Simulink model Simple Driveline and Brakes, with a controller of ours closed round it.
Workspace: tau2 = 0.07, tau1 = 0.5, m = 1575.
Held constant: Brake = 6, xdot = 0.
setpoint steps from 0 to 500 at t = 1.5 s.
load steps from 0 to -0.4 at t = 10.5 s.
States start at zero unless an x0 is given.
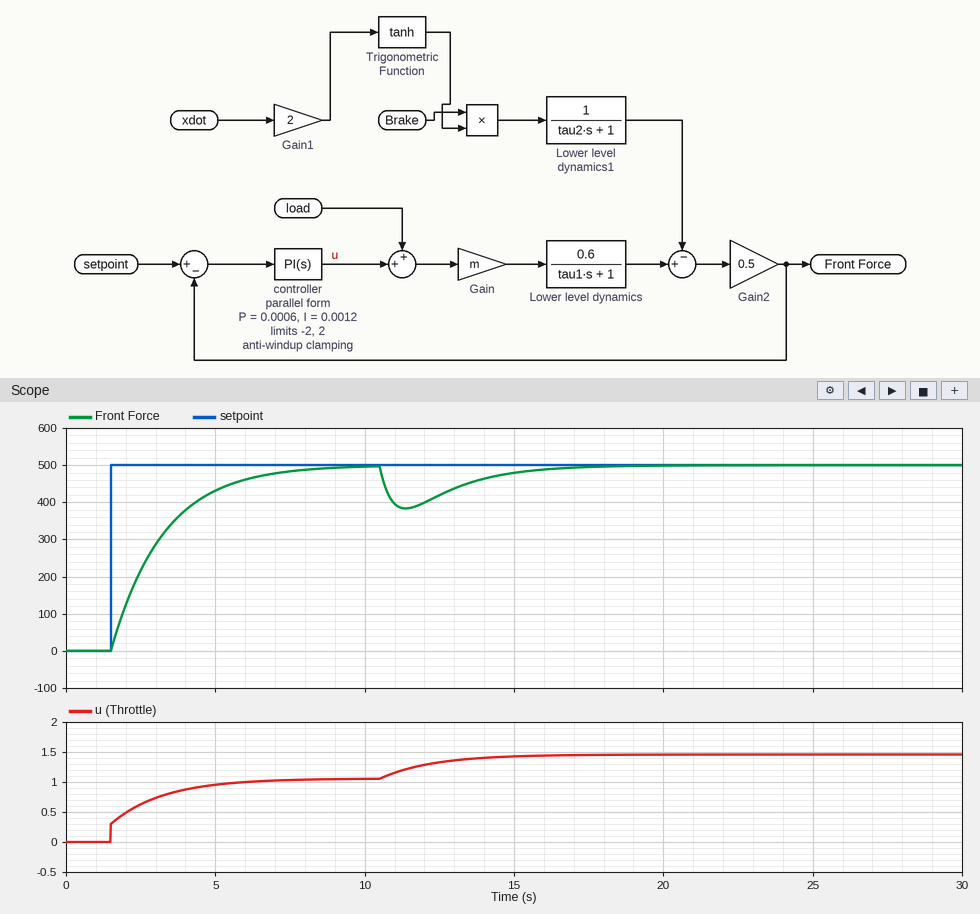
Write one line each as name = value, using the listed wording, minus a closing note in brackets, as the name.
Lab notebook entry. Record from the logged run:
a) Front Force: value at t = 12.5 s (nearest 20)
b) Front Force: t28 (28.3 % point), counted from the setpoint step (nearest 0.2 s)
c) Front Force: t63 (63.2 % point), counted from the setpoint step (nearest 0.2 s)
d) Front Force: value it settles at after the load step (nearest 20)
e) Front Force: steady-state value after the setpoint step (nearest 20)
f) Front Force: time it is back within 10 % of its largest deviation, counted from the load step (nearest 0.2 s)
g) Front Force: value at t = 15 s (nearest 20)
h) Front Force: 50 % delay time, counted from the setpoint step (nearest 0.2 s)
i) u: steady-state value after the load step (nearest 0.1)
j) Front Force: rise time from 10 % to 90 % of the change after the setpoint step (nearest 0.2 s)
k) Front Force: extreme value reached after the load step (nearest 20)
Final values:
Front Force: value at t = 12.5 s = 420
Front Force: t28 (28.3 % point), counted from the setpoint step = 0.6 s
Front Force: t63 (63.2 % point), counted from the setpoint step = 1.8 s
Front Force: value it settles at after the load step = 500
Front Force: steady-state value after the setpoint step = 500
Front Force: time it is back within 10 % of its largest deviation, counted from the load step = 5.6 s
Front Force: value at t = 15 s = 480
Front Force: 50 % delay time, counted from the setpoint step = 1.2 s
u: steady-state value after the load step = 1.5
Front Force: rise time from 10 % to 90 % of the change after the setpoint step = 3.8 s
Front Force: extreme value reached after the load step = 380
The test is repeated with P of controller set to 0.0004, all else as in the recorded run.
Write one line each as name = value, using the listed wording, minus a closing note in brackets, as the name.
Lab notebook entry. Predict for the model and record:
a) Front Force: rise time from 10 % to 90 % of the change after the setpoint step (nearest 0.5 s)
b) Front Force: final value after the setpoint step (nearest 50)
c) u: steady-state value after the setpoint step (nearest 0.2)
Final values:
Front Force: rise time from 10 % to 90 % of the change after the setpoint step = 3.5 s
Front Force: final value after the setpoint step = 500
u: steady-state value after the setpoint step = 1.0
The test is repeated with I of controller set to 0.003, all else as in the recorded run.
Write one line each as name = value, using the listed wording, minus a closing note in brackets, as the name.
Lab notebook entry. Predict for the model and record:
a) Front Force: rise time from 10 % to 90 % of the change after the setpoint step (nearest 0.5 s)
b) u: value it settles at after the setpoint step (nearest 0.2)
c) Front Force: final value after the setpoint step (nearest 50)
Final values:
Front Force: rise time from 10 % to 90 % of the change after the setpoint step = 1.5 s
u: value it settles at after the setpoint step = 1.0
Front Force: final value after the setpoint step = 500
